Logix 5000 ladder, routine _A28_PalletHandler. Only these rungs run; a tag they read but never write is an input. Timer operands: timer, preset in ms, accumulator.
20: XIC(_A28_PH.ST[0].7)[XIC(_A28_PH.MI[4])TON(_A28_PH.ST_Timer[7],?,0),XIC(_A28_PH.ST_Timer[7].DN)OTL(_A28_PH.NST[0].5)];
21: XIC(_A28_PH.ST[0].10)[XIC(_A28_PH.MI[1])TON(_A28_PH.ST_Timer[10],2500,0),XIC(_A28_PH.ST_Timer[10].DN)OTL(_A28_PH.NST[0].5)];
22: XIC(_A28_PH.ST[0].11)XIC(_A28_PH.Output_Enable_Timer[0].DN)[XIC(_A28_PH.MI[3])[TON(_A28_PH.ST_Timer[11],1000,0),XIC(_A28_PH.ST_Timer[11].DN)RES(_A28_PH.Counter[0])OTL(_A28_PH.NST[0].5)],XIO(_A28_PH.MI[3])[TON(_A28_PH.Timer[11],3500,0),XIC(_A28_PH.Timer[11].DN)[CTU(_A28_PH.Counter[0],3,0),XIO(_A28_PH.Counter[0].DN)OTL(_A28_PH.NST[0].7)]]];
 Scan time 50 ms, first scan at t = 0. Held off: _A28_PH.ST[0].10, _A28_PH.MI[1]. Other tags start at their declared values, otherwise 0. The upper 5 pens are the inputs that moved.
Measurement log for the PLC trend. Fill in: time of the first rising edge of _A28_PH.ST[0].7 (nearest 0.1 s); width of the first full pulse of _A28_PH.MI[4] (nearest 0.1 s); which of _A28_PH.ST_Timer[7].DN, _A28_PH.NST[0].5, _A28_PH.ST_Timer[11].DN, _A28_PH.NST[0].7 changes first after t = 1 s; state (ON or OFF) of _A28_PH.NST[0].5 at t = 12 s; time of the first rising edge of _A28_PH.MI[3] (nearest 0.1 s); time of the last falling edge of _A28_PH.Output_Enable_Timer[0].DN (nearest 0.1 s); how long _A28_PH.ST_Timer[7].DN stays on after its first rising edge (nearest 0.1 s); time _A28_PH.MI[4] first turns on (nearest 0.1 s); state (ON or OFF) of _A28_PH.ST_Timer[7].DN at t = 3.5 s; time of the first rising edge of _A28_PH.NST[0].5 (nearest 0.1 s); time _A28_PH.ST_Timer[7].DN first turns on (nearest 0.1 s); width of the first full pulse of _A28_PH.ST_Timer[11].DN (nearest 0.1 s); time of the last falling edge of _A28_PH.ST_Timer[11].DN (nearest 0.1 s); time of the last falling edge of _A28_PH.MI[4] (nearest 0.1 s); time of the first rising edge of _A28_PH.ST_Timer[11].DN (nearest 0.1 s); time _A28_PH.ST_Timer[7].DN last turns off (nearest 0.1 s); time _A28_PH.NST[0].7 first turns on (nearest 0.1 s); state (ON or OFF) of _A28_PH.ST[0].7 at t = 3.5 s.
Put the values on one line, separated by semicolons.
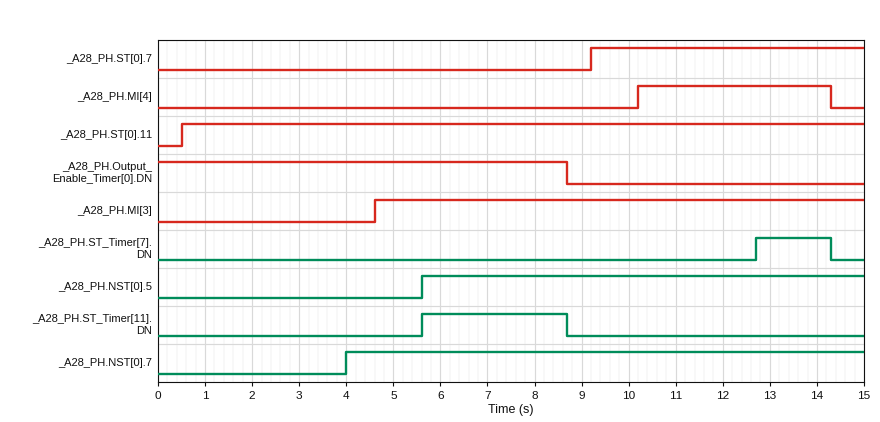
9.2 s; 4.1 s; _A28_PH.NST[0].7; ON; 4.6 s; 8.7 s; 1.6 s; 10.2 s; OFF; 5.6 s; 12.7 s; 3.1 s; 8.7 s; 14.3 s; 5.6 s; 14.3 s; 4.0 s; OFF
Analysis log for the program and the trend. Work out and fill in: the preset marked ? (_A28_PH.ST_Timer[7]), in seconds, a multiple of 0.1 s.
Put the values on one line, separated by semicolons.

2.5 s
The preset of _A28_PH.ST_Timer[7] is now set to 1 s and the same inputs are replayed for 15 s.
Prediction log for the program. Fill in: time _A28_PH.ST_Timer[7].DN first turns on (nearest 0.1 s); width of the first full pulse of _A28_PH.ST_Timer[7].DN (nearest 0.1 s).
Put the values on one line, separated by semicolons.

11.2 s; 3.1 s
